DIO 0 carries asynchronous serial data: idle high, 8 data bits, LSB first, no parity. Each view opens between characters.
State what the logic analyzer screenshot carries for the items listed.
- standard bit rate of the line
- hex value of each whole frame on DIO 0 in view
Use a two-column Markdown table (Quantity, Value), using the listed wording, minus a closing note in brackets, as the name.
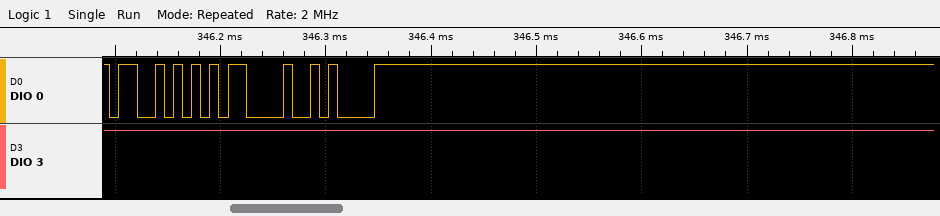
| Quantity | Value |
|---|---|
| standard bit rate of the line | 115200 baud |
| hex value of each whole frame on DIO 0 in view | 53, 0D, 0A |
